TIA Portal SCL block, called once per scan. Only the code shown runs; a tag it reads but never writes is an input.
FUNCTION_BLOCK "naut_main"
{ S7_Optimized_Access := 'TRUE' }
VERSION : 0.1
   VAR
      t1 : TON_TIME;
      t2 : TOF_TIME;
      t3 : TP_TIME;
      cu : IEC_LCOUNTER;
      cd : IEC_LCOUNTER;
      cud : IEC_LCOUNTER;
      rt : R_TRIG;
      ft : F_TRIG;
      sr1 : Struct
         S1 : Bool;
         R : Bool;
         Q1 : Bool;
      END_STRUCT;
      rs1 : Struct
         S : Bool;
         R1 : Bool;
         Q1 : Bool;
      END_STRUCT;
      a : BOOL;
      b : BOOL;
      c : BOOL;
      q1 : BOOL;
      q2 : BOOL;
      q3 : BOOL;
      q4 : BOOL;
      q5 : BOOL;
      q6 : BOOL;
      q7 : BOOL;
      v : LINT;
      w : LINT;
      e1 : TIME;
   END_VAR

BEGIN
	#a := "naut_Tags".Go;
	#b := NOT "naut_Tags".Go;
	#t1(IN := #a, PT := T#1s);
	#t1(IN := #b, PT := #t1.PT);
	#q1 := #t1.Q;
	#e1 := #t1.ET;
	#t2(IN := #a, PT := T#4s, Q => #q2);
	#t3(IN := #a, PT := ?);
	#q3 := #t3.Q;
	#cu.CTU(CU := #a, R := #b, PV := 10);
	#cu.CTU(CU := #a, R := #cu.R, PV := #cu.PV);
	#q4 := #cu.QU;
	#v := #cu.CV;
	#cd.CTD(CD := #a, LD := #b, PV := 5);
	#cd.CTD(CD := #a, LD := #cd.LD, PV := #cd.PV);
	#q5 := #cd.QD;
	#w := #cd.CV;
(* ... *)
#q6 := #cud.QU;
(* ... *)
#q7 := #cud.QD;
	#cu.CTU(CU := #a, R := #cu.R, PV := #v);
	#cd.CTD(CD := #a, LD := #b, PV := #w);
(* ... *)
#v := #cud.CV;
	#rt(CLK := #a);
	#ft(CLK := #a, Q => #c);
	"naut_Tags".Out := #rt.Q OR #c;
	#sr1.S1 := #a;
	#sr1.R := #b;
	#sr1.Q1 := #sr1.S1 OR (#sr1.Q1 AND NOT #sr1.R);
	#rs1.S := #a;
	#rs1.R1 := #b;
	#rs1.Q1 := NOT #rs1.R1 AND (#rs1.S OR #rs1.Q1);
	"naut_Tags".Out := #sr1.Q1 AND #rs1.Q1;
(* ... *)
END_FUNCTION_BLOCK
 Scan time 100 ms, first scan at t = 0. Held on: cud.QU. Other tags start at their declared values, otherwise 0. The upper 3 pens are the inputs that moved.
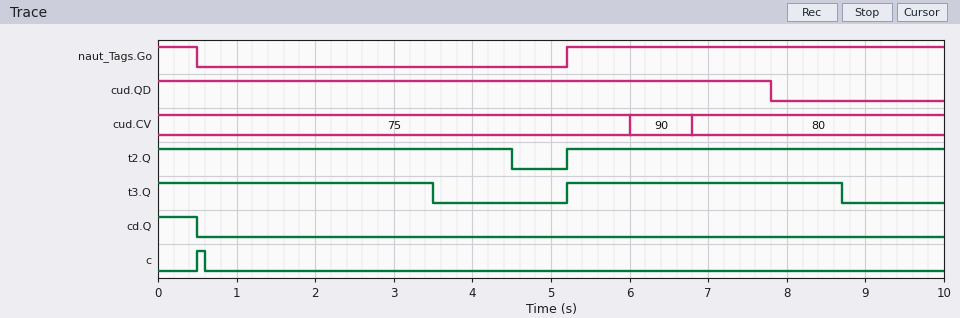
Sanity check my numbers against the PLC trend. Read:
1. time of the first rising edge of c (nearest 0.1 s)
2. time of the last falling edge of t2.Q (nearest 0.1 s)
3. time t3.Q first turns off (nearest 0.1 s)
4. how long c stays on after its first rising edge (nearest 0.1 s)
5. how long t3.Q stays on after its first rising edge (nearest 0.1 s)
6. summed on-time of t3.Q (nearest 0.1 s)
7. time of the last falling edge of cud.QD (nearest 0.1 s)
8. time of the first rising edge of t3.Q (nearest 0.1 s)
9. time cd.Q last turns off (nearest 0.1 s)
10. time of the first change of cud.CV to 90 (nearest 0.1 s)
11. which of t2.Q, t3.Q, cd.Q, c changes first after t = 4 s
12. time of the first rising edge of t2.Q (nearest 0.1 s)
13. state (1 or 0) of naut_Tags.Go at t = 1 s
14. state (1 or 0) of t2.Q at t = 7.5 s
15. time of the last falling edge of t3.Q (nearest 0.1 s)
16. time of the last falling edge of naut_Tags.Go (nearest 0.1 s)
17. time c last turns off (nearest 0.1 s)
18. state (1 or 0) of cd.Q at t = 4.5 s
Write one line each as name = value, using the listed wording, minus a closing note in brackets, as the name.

time of the first rising edge of c = 0.5 s
time of the last falling edge of t2.Q = 4.5 s
time t3.Q first turns off = 3.5 s
how long c stays on after its first rising edge = 0.1 s
how long t3.Q stays on after its first rising edge = 3.5 s
summed on-time of t3.Q = 7.0 s
time of the last falling edge of cud.QD = 7.8 s
time of the first rising edge of t3.Q = 5.2 s
time cd.Q last turns off = 0.5 s
time of the first change of cud.CV to 90 = 6.0 s
which of t2.Q, t3.Q, cd.Q, c changes first after t = 4 s = t2.Q
time of the first rising edge of t2.Q = 5.2 s
state (1 or 0) of naut_Tags.Go at t = 1 s = 0
state (1 or 0) of t2.Q at t = 7.5 s = 1
time of the last falling edge of t3.Q = 8.7 s
time of the last falling edge of naut_Tags.Go = 0.5 s
time c last turns off = 0.6 s
state (1 or 0) of cd.Q at t = 4.5 s = 0
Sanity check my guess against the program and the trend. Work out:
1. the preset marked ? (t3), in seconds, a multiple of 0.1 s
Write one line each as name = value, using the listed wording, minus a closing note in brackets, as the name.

the preset marked ? (t3), in seconds, a multiple of 0.1 s = 3.5 s
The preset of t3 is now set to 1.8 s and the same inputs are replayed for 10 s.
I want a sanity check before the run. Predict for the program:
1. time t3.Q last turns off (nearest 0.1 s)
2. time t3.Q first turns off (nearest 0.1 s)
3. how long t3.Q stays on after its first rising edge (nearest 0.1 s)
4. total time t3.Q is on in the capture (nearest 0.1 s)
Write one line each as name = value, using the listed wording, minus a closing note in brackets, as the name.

time t3.Q last turns off = 7.0 s
time t3.Q first turns off = 1.8 s
how long t3.Q stays on after its first rising edge = 1.8 s
total time t3.Q is on in the capture = 3.6 s
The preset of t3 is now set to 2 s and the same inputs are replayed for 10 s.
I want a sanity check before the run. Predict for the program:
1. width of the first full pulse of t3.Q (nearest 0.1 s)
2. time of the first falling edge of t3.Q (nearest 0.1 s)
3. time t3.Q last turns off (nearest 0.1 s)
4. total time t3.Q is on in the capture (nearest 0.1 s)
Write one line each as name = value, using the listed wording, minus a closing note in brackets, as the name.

width of the first full pulse of t3.Q = 2.0 s
time of the first falling edge of t3.Q = 2.0 s
time t3.Q last turns off = 7.2 s
total time t3.Q is on in the capture = 4.0 s
